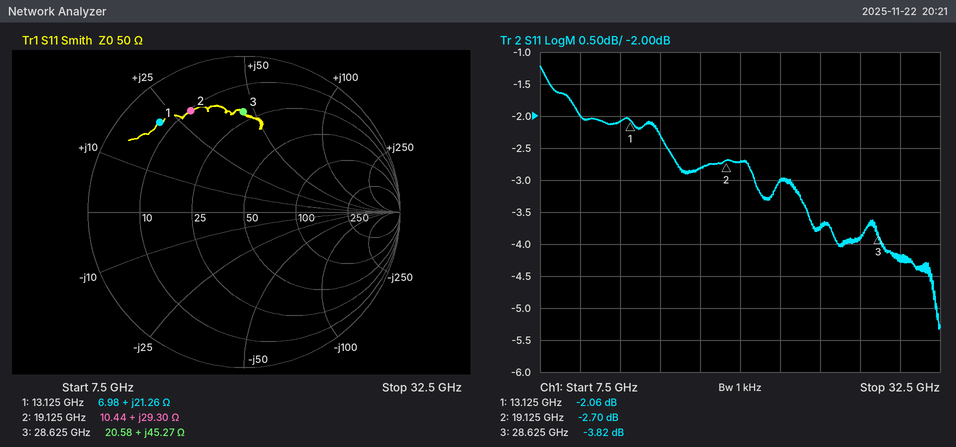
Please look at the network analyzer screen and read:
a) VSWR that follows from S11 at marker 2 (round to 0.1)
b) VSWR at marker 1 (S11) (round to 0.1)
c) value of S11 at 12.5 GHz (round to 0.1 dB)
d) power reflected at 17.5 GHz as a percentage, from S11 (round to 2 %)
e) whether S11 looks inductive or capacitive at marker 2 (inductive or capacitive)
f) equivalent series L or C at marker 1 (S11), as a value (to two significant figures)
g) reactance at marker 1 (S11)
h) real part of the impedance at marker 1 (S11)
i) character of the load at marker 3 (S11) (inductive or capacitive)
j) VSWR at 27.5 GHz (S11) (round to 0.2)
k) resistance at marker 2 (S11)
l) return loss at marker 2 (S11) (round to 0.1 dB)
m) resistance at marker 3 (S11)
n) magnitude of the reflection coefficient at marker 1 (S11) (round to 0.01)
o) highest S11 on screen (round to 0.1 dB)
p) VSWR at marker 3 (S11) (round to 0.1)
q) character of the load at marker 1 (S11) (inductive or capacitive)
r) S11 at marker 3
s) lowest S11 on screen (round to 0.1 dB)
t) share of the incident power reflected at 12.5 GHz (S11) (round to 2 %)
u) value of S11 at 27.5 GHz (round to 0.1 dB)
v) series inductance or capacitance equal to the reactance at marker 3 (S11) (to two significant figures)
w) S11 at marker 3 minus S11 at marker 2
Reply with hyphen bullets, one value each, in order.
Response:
- 6.5
- 8.5
- -2.1 dB
- 52 %
- inductive
- 260 pH
- +21.26 Ω
- 6.98 Ω
- inductive
- 4.6
- 10.44 Ω
- 2.7 dB
- 20.58 Ω
- 0.79
- -1.2 dB
- 4.6
- inductive
- -3.82 dB
- -5.3 dB
- 62 %
- -3.9 dB
- 250 pH
- -1.12 dB
